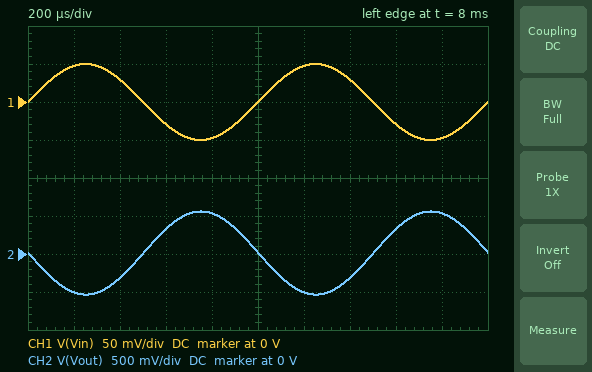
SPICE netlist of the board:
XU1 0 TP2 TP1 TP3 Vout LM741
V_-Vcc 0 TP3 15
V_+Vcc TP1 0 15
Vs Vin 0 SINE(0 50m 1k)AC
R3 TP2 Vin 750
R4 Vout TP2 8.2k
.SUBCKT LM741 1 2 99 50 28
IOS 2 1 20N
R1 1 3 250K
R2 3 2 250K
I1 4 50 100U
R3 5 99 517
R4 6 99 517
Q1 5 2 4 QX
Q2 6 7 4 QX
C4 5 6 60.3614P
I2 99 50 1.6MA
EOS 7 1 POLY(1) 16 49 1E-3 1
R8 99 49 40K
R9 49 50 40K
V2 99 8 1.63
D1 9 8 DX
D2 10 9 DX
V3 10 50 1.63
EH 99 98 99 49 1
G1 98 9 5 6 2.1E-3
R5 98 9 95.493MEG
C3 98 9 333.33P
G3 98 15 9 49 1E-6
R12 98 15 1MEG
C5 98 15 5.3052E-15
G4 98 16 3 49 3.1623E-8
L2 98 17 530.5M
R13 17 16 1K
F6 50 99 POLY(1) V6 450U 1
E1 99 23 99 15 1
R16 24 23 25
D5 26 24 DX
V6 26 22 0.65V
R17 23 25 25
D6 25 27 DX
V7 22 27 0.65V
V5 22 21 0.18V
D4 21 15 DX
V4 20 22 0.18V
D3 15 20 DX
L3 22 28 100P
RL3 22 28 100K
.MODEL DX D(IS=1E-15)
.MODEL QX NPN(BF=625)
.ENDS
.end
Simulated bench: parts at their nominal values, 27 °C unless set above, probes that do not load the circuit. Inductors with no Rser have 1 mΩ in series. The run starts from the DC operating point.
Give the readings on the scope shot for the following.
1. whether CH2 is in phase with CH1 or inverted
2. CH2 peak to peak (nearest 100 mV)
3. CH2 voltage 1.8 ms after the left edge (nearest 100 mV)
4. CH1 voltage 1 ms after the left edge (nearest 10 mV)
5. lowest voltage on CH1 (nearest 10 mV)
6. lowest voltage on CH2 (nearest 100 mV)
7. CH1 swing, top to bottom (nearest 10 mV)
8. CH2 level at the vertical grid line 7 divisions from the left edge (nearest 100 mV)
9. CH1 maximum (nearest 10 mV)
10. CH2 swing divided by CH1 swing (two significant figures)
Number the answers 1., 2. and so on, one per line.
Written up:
1. inverted
2. 1.1 V
3. 500 mV
4. 0 V
5. -50 mV
6. -500 mV
7. 100 mV
8. -300 mV
9. 50 mV
10. 11
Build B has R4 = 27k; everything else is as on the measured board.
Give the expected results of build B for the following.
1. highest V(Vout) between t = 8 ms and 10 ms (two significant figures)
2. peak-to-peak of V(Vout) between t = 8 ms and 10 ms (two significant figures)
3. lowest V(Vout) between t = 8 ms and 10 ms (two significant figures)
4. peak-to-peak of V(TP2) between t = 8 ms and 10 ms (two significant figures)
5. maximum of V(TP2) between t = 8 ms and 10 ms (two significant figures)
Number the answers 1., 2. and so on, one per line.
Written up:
1. 1.8 V
2. 3.6 V
3. -1.8 V
4. 3.6 mV
5. 2.8 mV
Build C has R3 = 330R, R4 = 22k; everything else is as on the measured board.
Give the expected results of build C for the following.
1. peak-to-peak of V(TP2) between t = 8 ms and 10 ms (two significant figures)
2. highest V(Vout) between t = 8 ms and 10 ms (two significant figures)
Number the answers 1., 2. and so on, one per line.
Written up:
1. 6.7 mV
2. 3.4 V
